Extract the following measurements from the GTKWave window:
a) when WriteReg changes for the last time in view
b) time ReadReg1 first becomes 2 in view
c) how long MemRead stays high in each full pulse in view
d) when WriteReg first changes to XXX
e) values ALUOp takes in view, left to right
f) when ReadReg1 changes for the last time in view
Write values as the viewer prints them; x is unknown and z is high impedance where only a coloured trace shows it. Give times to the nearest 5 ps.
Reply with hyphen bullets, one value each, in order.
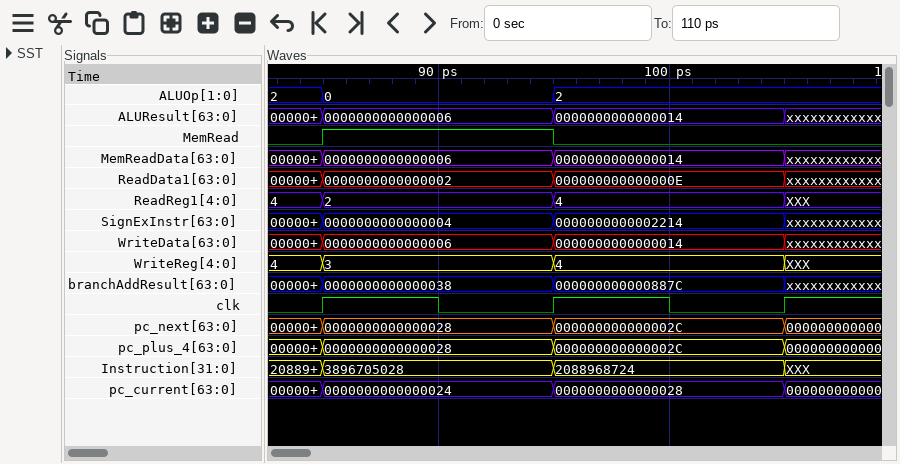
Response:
- 105 ps
- 85 ps
- 10 ps
- 105 ps
- 2, 0, 2
- 105 ps
